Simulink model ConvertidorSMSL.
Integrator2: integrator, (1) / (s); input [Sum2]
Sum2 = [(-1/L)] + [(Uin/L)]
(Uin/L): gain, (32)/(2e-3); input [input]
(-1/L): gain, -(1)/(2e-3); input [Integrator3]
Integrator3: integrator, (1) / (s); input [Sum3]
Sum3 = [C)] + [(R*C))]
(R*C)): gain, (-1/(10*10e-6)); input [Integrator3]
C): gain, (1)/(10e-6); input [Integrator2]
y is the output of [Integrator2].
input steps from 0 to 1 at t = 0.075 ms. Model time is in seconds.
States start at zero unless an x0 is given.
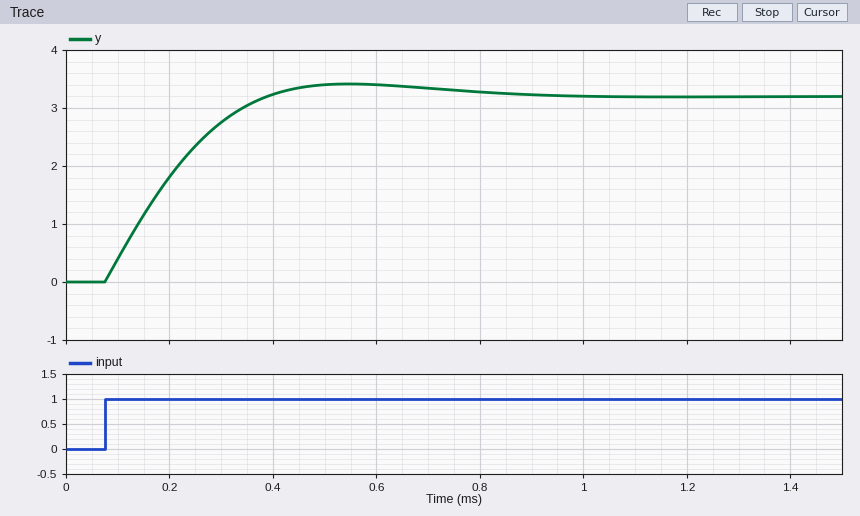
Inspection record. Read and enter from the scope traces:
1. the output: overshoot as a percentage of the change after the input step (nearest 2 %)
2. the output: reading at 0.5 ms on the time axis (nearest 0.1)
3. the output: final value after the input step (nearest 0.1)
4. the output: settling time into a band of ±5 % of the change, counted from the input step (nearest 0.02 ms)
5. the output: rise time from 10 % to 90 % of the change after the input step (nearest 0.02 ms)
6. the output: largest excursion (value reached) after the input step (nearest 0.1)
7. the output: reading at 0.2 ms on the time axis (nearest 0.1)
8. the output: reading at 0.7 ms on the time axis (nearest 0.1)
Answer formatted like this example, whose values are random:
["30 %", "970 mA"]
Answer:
["6 %", "3.4", "3.2", "0.60 ms", "0.22 ms", "3.4", "1.8", "3.3"]
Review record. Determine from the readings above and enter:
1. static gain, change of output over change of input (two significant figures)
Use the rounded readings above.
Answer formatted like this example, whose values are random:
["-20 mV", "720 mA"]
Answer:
["3.2"]
